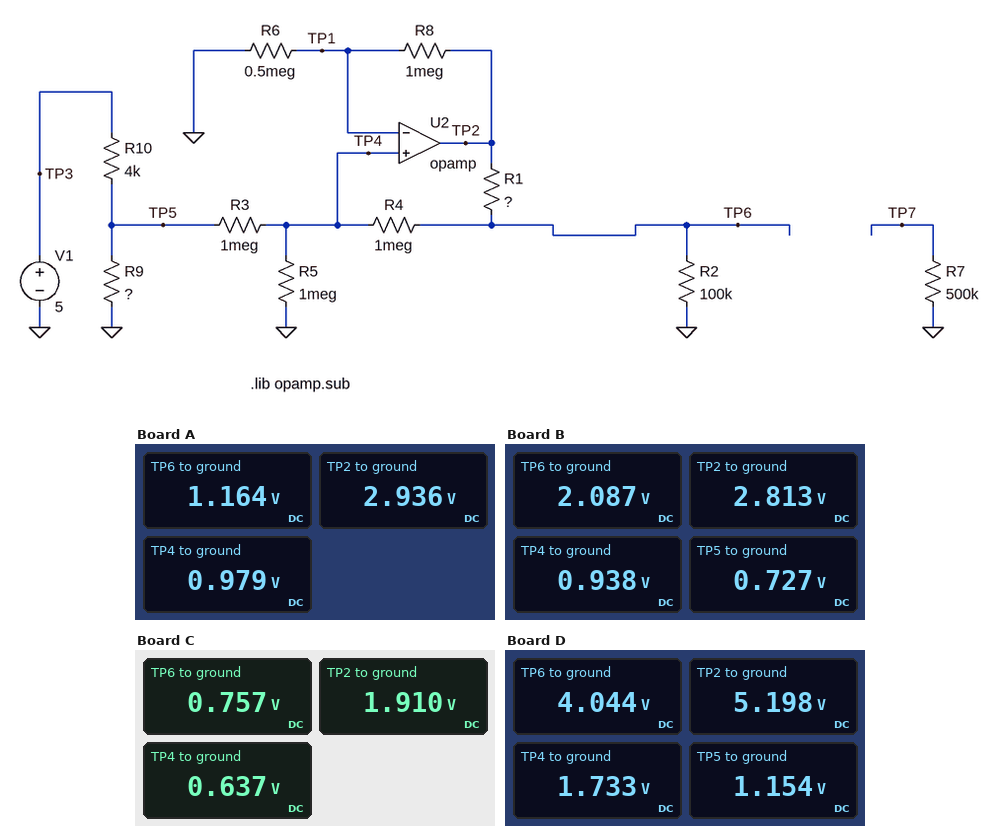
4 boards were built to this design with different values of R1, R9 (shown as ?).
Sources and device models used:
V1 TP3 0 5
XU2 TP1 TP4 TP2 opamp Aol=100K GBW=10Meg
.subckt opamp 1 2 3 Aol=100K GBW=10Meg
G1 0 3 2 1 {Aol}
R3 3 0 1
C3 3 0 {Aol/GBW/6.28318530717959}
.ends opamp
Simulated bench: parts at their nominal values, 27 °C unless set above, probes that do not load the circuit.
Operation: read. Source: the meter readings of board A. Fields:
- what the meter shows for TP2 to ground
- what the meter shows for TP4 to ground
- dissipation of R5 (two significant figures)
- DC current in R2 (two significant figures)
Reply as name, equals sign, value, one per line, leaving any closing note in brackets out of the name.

what the meter shows for TP2 to ground = 2.936 V
what the meter shows for TP4 to ground = 0.979 V
dissipation of R5 = 960 nW
DC current in R2 = 12 µA
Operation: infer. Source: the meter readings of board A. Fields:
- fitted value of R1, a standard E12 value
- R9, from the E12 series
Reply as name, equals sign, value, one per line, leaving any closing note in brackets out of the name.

fitted value of R1, a standard E12 value = 150 kΩ
R9, from the E12 series = 2.2 kΩ
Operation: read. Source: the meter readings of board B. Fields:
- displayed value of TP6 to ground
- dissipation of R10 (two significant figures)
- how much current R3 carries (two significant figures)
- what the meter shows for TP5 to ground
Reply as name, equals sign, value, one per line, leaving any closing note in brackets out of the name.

displayed value of TP6 to ground = 2.087 V
dissipation of R10 = 4.6 mW
how much current R3 carries = 210 nA
what the meter shows for TP5 to ground = 0.727 V
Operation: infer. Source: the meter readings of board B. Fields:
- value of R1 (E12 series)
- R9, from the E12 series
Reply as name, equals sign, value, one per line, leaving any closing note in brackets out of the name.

value of R1 = 33 kΩ
R9, from the E12 series = 680 Ω
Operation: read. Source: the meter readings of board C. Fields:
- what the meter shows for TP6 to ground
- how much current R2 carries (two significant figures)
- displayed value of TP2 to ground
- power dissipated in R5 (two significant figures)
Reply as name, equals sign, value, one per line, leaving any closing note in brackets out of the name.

what the meter shows for TP6 to ground = 0.757 V
how much current R2 carries = 7.6 µA
displayed value of TP2 to ground = 1.910 V
power dissipated in R5 = 410 nW
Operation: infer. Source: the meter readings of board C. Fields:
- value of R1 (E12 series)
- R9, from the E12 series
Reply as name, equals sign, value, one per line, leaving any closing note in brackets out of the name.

value of R1 = 150 kΩ
R9, from the E12 series = 1.2 kΩ
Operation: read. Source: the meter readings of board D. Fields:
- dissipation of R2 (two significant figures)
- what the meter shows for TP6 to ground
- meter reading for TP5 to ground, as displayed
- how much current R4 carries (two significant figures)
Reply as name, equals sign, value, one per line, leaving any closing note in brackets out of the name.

dissipation of R2 = 160 µW
what the meter shows for TP6 to ground = 4.044 V
meter reading for TP5 to ground, as displayed = 1.154 V
how much current R4 carries = 2.3 µA
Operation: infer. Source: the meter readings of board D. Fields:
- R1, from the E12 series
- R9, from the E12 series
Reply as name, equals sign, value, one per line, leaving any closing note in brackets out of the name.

R1, from the E12 series = 27 kΩ
R9, from the E12 series = 1.2 kΩ
